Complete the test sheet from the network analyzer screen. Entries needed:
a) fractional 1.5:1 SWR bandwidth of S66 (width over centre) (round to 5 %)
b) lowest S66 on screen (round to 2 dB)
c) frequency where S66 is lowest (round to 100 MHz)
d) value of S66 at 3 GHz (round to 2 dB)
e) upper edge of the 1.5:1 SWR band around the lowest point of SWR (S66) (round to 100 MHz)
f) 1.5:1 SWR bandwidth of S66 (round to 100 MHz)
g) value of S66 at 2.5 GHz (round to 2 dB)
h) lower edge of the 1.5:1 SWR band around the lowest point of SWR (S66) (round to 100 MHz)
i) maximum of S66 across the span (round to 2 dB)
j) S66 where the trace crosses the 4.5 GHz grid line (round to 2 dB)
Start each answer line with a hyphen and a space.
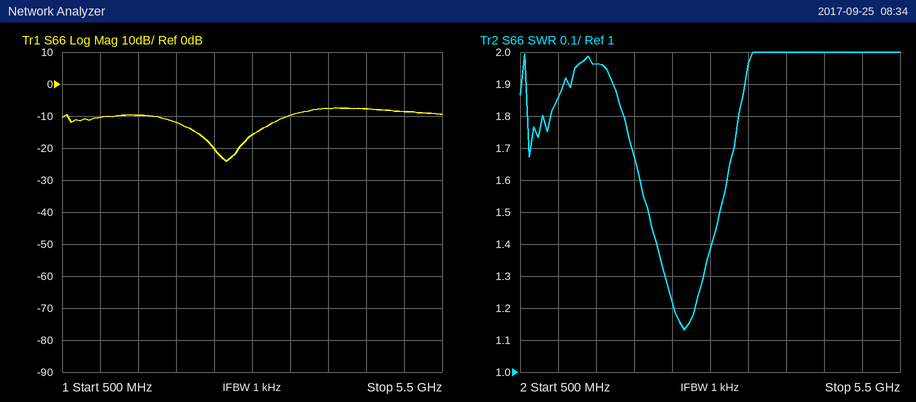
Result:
- 35 %
- -24 dB
- 2.7 GHz
- -16 dB
- 3.1 GHz
- 900 MHz
- -20 dB
- 2.2 GHz
- -8 dB
- -8 dB
